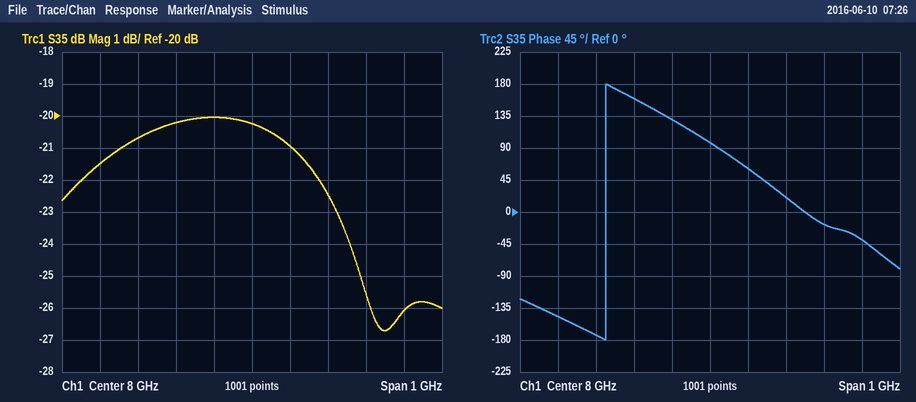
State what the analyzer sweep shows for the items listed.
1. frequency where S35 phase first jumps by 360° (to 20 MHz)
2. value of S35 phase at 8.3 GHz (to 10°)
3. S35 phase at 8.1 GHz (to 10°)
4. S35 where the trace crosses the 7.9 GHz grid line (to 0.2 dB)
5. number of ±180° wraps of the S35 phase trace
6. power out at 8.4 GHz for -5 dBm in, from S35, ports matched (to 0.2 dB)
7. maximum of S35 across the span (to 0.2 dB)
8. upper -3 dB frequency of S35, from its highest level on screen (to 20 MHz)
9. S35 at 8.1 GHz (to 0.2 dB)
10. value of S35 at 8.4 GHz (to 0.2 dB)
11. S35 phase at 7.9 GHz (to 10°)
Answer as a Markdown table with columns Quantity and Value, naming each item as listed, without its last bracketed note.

| Quantity | Value |
|---|---|
| frequency where S35 phase first jumps by 360° | 7.72 GHz |
| value of S35 phase at 8.3 GHz | -20° |
| S35 phase at 8.1 GHz | 60° |
| S35 where the trace crosses the 7.9 GHz grid line | -20.0 dB |
| number of ±180° wraps of the S35 phase trace | 1 |
| power out at 8.4 GHz for -5 dBm in, from S35, ports matched | -31.0 dBm |
| maximum of S35 across the span | -20.0 dB |
| upper -3 dB frequency of S35, from its highest level on screen | 8.22 GHz |
| S35 at 8.1 GHz | -21.0 dB |
| value of S35 at 8.4 GHz | -26.0 dB |
| S35 phase at 7.9 GHz | 130° |
